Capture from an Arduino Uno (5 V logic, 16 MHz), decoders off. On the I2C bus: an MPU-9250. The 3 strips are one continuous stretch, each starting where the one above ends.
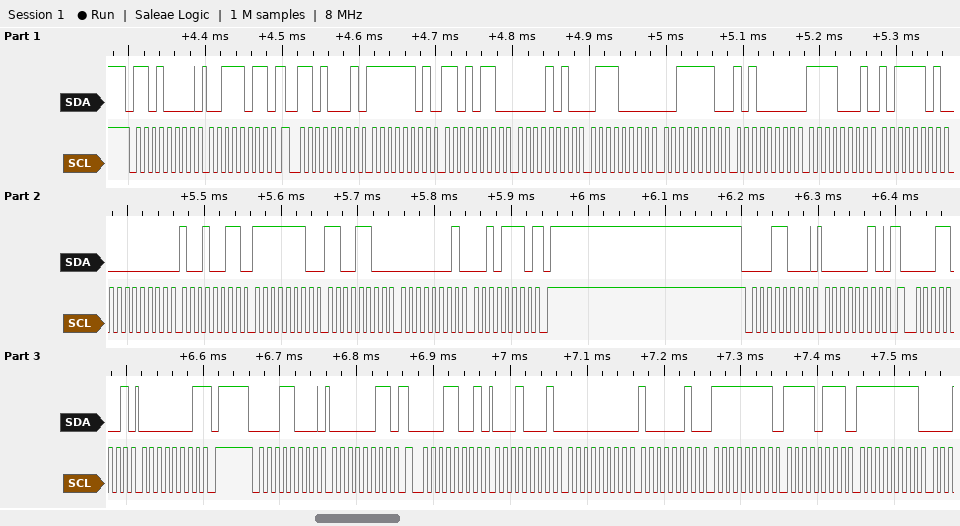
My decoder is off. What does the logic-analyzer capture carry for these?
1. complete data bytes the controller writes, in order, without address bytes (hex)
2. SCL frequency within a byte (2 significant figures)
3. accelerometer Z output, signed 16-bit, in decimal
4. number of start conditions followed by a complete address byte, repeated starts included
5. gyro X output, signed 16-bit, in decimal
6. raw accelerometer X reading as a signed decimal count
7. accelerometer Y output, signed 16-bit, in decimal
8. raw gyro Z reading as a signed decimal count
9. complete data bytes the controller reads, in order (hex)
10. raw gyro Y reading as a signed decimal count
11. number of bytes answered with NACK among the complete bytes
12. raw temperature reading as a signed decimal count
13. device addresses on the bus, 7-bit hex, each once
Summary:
3B 02 03
100 kHz
16032
6
147
-554
2672
302
FD D6 0A 70 3E A0 F1 BD 00 93 FE CC 01 2E 01 11 00 82 FF F7 FF
-308
2
-3651
0x68 0x0C
